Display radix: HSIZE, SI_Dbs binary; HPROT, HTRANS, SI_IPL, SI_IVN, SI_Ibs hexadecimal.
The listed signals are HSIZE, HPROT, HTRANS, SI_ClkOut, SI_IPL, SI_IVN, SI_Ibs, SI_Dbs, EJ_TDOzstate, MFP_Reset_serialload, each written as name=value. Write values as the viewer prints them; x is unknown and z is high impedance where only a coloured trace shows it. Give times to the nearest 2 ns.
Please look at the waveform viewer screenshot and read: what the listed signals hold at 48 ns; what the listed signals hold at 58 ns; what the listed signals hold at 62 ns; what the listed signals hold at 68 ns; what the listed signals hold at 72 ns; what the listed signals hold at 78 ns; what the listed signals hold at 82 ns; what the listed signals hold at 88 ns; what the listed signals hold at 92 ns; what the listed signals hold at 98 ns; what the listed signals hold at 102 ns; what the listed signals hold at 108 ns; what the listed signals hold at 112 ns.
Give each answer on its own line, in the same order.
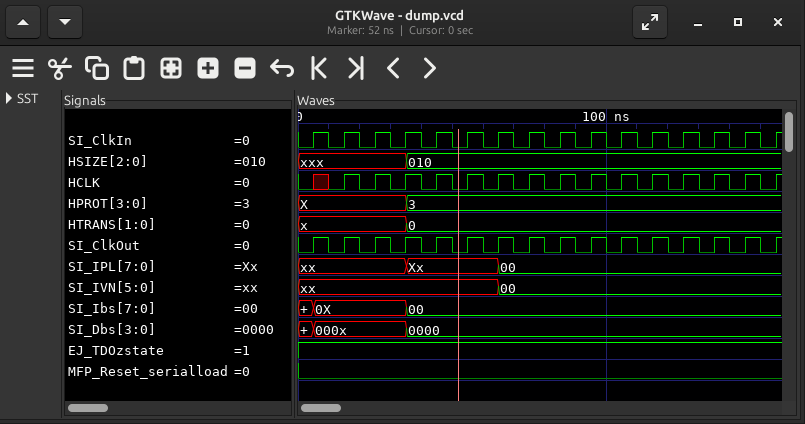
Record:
HSIZE=010, HPROT=3, HTRANS=0, SI_ClkOut=1, SI_IPL=Xx, SI_IVN=xx, SI_Ibs=00, SI_Dbs=0000, EJ_TDOzstate=1, MFP_Reset_serialload=0
HSIZE=010, HPROT=3, HTRANS=0, SI_ClkOut=1, SI_IPL=Xx, SI_IVN=xx, SI_Ibs=00, SI_Dbs=0000, EJ_TDOzstate=1, MFP_Reset_serialload=0
HSIZE=010, HPROT=3, HTRANS=0, SI_ClkOut=0, SI_IPL=Xx, SI_IVN=xx, SI_Ibs=00, SI_Dbs=0000, EJ_TDOzstate=1, MFP_Reset_serialload=0
HSIZE=010, HPROT=3, HTRANS=0, SI_ClkOut=1, SI_IPL=00, SI_IVN=00, SI_Ibs=00, SI_Dbs=0000, EJ_TDOzstate=1, MFP_Reset_serialload=0
HSIZE=010, HPROT=3, HTRANS=0, SI_ClkOut=0, SI_IPL=00, SI_IVN=00, SI_Ibs=00, SI_Dbs=0000, EJ_TDOzstate=1, MFP_Reset_serialload=0
HSIZE=010, HPROT=3, HTRANS=0, SI_ClkOut=1, SI_IPL=00, SI_IVN=00, SI_Ibs=00, SI_Dbs=0000, EJ_TDOzstate=1, MFP_Reset_serialload=0
HSIZE=010, HPROT=3, HTRANS=0, SI_ClkOut=0, SI_IPL=00, SI_IVN=00, SI_Ibs=00, SI_Dbs=0000, EJ_TDOzstate=1, MFP_Reset_serialload=0
HSIZE=010, HPROT=3, HTRANS=0, SI_ClkOut=1, SI_IPL=00, SI_IVN=00, SI_Ibs=00, SI_Dbs=0000, EJ_TDOzstate=1, MFP_Reset_serialload=0
HSIZE=010, HPROT=3, HTRANS=0, SI_ClkOut=0, SI_IPL=00, SI_IVN=00, SI_Ibs=00, SI_Dbs=0000, EJ_TDOzstate=1, MFP_Reset_serialload=0
HSIZE=010, HPROT=3, HTRANS=0, SI_ClkOut=1, SI_IPL=00, SI_IVN=00, SI_Ibs=00, SI_Dbs=0000, EJ_TDOzstate=1, MFP_Reset_serialload=0
HSIZE=010, HPROT=3, HTRANS=0, SI_ClkOut=0, SI_IPL=00, SI_IVN=00, SI_Ibs=00, SI_Dbs=0000, EJ_TDOzstate=1, MFP_Reset_serialload=0
HSIZE=010, HPROT=3, HTRANS=0, SI_ClkOut=1, SI_IPL=00, SI_IVN=00, SI_Ibs=00, SI_Dbs=0000, EJ_TDOzstate=1, MFP_Reset_serialload=0
HSIZE=010, HPROT=3, HTRANS=0, SI_ClkOut=0, SI_IPL=00, SI_IVN=00, SI_Ibs=00, SI_Dbs=0000, EJ_TDOzstate=1, MFP_Reset_serialload=0
